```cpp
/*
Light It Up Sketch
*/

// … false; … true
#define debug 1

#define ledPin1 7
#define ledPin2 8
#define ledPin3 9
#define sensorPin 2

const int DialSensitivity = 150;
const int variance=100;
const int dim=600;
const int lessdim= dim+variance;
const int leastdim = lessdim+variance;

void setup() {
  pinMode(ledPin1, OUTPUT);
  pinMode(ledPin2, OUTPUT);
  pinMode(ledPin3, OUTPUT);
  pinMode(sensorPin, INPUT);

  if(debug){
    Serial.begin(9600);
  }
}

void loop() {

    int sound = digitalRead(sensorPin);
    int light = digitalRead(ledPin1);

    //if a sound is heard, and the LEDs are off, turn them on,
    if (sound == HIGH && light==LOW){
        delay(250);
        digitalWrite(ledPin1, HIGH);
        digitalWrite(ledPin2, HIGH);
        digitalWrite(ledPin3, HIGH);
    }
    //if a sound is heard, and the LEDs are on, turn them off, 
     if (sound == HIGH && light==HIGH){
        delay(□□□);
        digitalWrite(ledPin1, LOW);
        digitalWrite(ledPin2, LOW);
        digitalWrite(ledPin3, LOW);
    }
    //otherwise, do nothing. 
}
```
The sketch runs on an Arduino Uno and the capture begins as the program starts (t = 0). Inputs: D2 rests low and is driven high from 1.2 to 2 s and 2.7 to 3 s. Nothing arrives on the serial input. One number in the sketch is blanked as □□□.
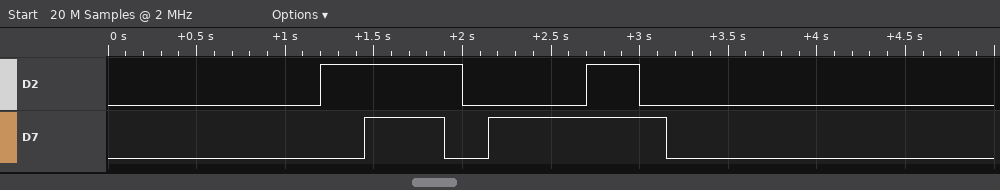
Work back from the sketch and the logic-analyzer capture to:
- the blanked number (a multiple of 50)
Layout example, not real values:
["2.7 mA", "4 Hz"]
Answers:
["450"]
